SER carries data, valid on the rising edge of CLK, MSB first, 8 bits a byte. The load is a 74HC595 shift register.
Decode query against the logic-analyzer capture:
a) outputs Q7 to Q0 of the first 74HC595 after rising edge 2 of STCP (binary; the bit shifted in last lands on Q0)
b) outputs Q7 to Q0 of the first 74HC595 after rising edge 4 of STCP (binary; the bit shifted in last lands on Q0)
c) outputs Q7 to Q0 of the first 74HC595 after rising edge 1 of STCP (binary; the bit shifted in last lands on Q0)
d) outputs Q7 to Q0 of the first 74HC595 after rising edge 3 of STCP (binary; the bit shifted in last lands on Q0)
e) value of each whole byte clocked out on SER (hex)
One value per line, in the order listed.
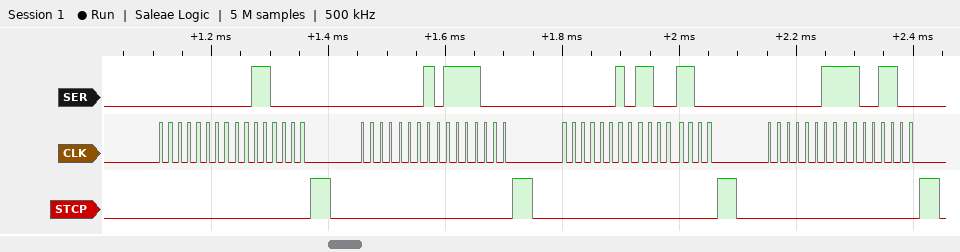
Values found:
01111000
11001100
00110000
11001100
0x00 0x30 0x01 0x78 0x02 0xCC 0x03 0xCC
